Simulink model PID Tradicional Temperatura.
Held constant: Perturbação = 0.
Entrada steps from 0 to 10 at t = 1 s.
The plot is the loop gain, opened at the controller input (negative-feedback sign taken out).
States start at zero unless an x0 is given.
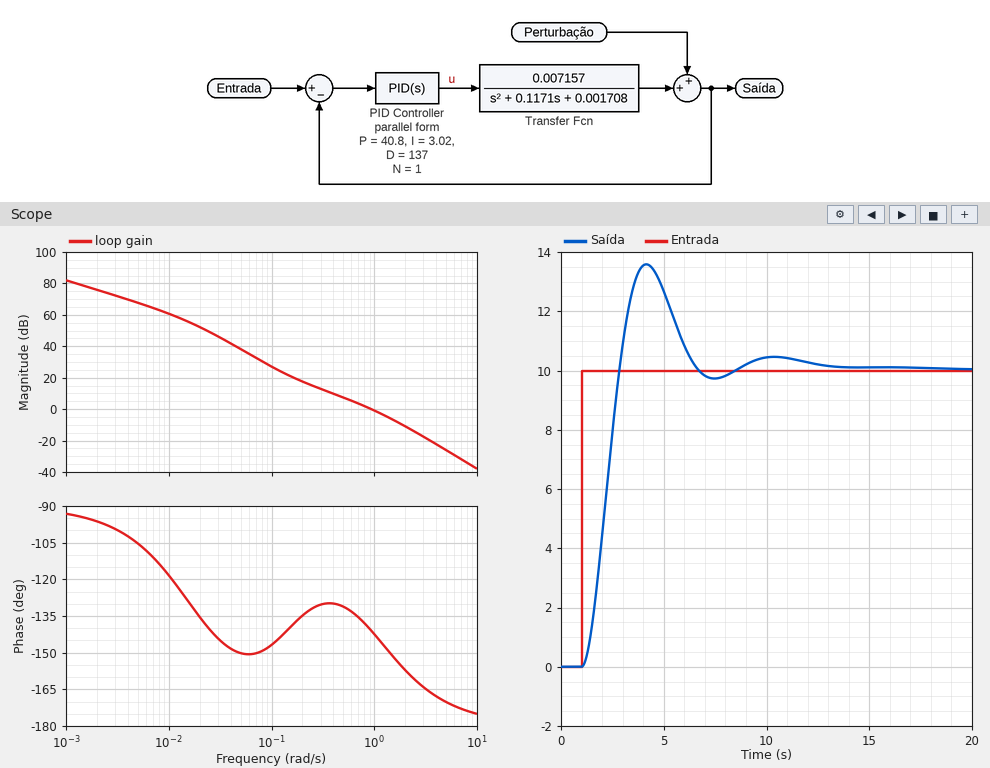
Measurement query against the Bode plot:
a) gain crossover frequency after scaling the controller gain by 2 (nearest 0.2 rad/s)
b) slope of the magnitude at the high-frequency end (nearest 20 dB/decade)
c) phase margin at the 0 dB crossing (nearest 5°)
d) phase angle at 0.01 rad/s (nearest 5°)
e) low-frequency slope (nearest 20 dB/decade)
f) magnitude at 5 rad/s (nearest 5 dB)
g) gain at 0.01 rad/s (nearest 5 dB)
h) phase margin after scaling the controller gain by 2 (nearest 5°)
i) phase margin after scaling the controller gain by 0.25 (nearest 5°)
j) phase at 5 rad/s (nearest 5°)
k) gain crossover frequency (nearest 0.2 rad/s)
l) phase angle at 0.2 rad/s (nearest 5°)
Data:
1.4 rad/s
-40 dB/decade
40°
-120°
-20 dB/decade
-25 dB
60 dB
30°
50°
-170°
1.0 rad/s
-135°
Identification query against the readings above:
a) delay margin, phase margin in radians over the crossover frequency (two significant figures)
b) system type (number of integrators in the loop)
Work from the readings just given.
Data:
0.70 s
1
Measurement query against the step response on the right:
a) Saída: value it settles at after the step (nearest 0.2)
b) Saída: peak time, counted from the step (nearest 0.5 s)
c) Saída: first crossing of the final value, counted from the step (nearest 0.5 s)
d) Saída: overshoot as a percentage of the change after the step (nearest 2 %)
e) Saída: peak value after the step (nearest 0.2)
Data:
10.0
3.0 s
2.0 s
36 %
13.6
